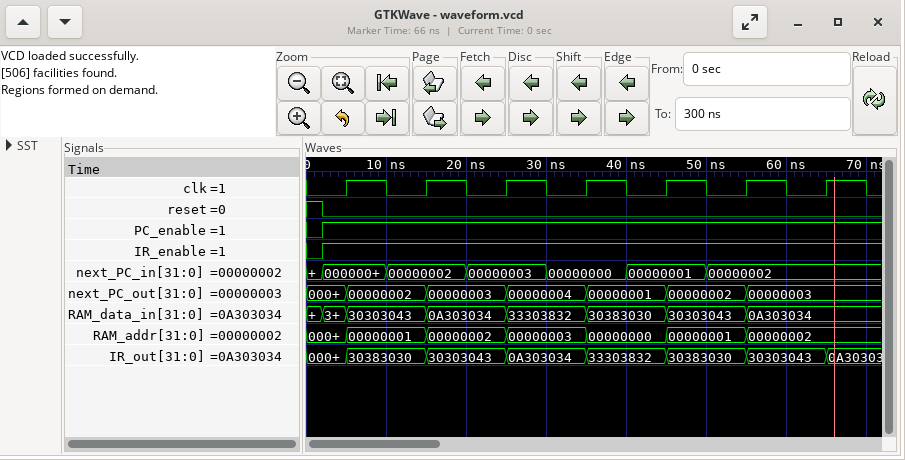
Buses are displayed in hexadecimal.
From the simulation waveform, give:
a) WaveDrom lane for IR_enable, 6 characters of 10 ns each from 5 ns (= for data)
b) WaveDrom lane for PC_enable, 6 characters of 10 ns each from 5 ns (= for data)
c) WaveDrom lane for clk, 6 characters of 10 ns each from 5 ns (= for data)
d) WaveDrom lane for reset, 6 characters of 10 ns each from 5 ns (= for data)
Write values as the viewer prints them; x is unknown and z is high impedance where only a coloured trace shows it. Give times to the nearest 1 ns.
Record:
{name: 'IR_enable', wave: '1.....'}
{name: 'PC_enable', wave: '1.....'}
{name: 'clk', wave: 'p.....'}
{name: 'reset', wave: '0.....'}
